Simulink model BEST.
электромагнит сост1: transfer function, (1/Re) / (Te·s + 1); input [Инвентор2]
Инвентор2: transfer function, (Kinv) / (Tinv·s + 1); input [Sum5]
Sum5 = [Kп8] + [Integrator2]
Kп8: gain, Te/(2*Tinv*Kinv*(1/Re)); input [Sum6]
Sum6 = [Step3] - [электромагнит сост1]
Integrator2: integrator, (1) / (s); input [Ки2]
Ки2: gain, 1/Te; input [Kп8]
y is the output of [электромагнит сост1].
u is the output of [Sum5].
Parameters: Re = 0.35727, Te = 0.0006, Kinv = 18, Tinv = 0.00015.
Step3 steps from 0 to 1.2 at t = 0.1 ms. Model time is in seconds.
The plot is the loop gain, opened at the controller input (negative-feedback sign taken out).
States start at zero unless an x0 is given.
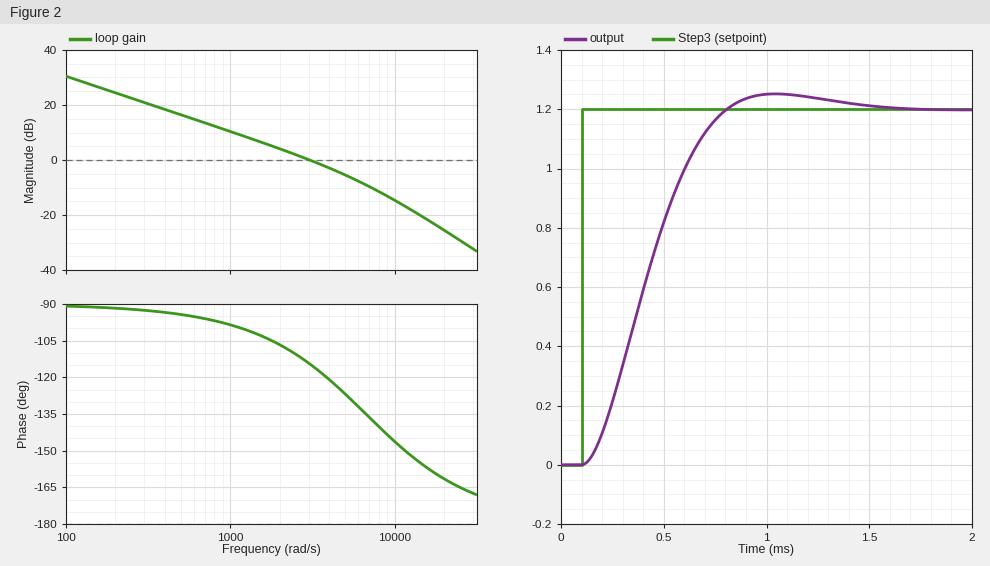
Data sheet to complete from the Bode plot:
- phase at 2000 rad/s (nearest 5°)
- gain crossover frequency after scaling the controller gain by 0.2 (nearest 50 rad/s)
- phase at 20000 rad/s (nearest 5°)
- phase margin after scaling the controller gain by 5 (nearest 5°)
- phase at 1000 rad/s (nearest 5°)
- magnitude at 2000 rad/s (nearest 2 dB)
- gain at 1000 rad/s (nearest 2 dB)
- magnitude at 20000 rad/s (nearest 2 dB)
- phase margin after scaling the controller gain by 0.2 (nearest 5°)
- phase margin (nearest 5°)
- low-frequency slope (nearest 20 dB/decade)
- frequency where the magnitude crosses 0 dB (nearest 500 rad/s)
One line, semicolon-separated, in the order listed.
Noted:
-105°; 650 rad/s; -160°; 35°; -100°; 4 dB; 10 dB; -26 dB; 85°; 65°; -20 dB/decade; 3000 rad/s
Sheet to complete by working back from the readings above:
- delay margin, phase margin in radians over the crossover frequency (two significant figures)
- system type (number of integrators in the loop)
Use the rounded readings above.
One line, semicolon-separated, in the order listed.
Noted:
0.00038 s; 1
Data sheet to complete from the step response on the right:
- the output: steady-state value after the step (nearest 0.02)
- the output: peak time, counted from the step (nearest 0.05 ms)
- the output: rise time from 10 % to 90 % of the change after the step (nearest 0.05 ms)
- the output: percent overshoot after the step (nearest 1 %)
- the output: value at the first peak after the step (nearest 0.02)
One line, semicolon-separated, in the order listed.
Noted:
1.20; 0.95 ms; 0.45 ms; 4 %; 1.26
